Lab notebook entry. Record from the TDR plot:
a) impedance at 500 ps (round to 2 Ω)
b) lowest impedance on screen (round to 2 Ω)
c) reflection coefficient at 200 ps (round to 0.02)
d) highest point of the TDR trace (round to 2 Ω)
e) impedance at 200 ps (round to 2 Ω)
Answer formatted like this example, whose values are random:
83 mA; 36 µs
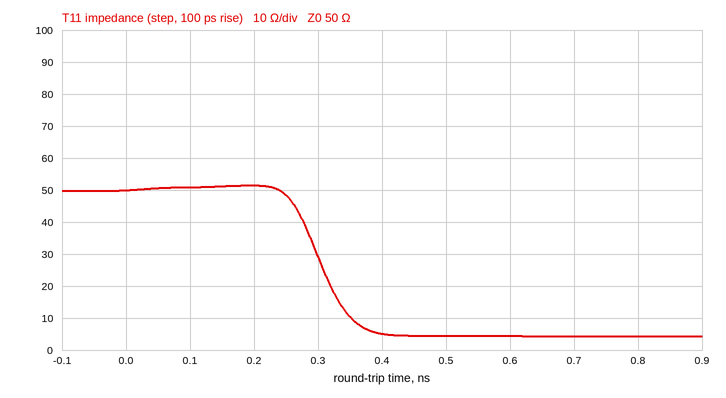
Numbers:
4 Ω; 4 Ω; +0.02; 52 Ω; 52 Ω
